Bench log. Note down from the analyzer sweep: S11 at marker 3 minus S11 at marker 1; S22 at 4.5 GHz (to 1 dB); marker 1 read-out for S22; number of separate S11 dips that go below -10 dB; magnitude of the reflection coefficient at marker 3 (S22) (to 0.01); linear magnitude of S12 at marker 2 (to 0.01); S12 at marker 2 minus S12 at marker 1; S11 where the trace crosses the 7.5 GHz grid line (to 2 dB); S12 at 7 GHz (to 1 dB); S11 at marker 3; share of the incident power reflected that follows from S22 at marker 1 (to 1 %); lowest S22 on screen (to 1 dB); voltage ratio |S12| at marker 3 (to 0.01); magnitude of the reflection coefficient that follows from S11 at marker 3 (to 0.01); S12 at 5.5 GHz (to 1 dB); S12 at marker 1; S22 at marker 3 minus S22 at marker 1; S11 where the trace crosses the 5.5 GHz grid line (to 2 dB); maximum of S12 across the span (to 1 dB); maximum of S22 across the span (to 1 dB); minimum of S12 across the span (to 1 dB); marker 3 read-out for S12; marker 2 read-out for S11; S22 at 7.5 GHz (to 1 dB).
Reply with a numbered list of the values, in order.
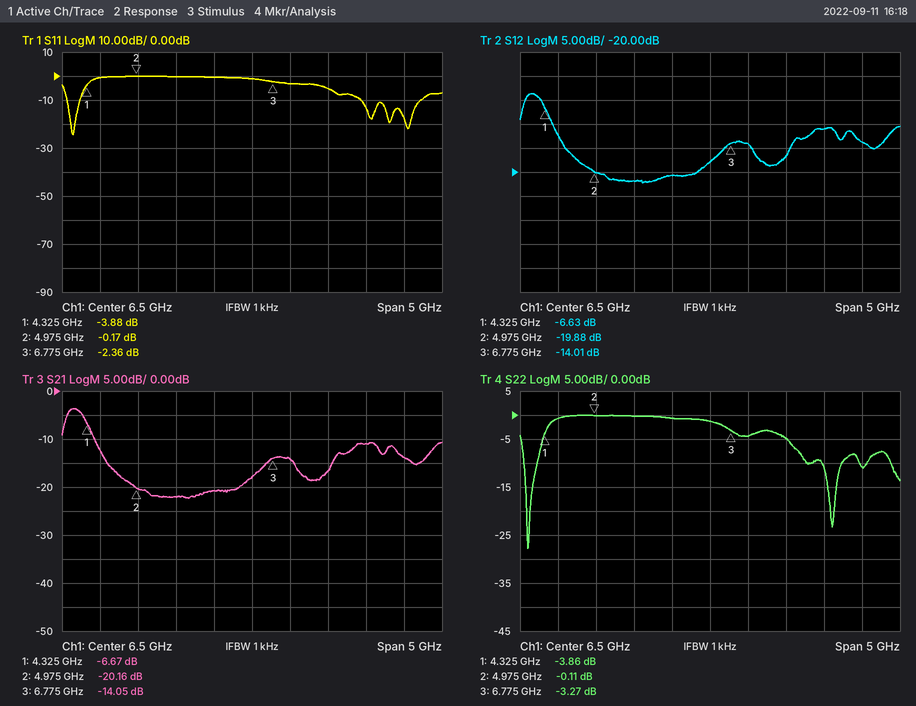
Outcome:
1. 1.52 dB
2. -1 dB
3. -3.86 dB
4. 4
5. 0.69
6. 0.10
7. -13.25 dB
8. -6 dB
9. -14 dB
10. -2.36 dB
11. 41 %
12. -28 dB
13. 0.20
14. 0.76
15. -22 dB
16. -6.63 dB
17. 0.59 dB
18. 0 dB
19. -4 dB
20. 0 dB
21. -22 dB
22. -14.01 dB
23. -0.17 dB
24. -5 dB
